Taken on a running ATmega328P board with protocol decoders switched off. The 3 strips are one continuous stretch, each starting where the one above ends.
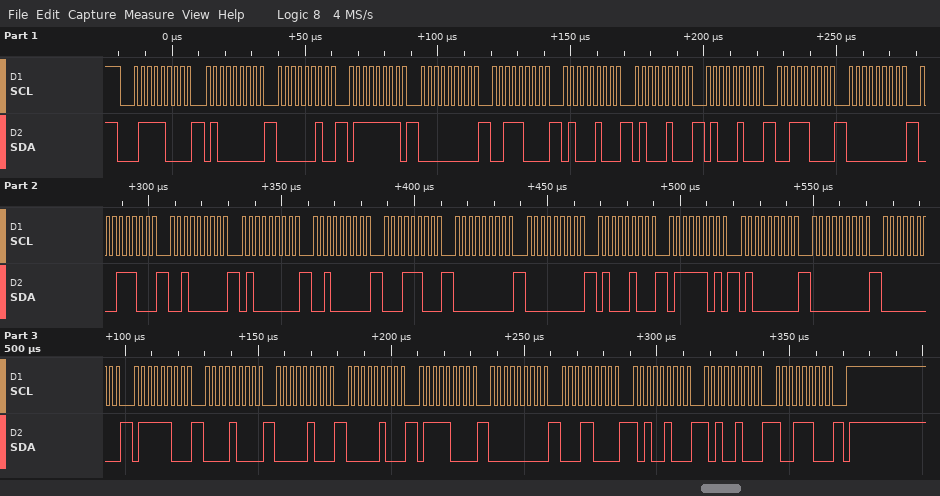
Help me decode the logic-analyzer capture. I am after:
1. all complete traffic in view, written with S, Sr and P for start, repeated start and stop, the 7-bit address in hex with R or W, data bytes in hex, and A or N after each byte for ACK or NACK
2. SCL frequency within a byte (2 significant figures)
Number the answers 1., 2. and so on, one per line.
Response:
1. S 3CW A 40 A 02 A 7F A 00 A 38 A 44 A 44 A 44 A 38 A 00 A 1C A 20 A 40 A 20 A 1C A 00 A 00 A 44 A 7D A 40 A 00 A 00 A 7C A 08 A 04 A 04 A 78 A 00 A 18 A A4 A A4 A 9C A P
2. 400 kHz
